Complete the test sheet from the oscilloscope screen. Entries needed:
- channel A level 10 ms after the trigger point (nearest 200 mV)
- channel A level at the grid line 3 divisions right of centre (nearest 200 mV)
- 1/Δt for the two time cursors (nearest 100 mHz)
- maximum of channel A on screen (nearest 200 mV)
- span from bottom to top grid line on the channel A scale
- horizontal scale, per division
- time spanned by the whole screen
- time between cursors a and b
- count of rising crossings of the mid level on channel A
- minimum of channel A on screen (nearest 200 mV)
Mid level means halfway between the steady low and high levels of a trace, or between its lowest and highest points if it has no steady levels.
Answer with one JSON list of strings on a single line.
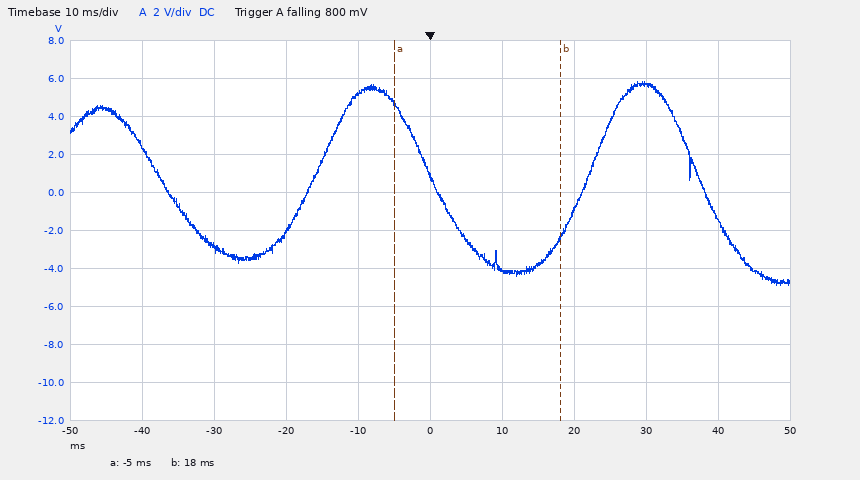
["-4.0 V", "5.6 V", "43.5 Hz", "5.8 V", "20 V", "10 ms", "100 ms", "23 ms", "2", "-4.8 V"]
